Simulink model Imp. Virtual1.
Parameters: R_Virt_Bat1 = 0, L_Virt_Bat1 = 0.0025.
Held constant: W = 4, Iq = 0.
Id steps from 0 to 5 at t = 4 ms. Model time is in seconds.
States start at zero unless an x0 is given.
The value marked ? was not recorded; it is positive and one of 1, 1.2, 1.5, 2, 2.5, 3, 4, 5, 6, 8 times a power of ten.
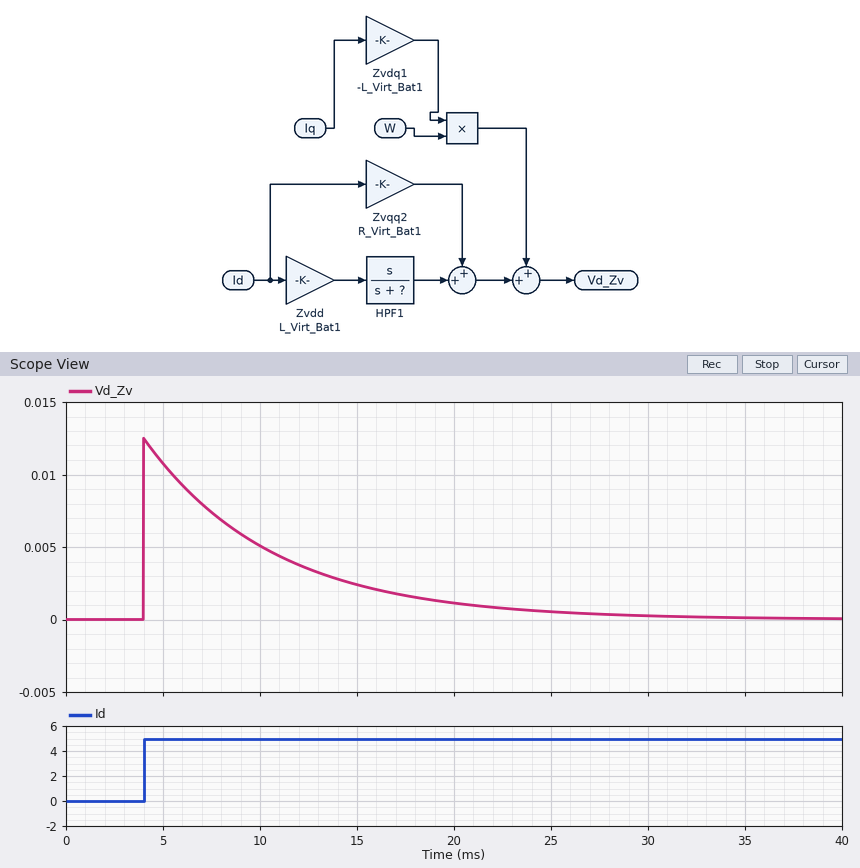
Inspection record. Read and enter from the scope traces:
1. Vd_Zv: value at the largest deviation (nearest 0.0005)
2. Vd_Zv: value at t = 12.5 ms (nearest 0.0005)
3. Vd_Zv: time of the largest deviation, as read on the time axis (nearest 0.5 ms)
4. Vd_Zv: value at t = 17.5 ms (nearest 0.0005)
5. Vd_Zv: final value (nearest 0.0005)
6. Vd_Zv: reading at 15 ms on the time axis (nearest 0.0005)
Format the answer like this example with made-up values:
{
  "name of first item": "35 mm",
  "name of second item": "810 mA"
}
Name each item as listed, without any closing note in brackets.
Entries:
{
  "Vd_Zv: value at the largest deviation": "0.0125",
  "Vd_Zv: value at t = 12.5 ms": "0.0035",
  "Vd_Zv: time of the largest deviation, as read on the time axis": "4.0 ms",
  "Vd_Zv: value at t = 17.5 ms": "0.0015",
  "Vd_Zv: final value": "0.0000",
  "Vd_Zv: reading at 15 ms on the time axis": "0.0025"
}
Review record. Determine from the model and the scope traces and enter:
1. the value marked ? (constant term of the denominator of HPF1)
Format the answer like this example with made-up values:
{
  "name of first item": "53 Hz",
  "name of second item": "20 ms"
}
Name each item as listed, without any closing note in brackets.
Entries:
{
  "the value marked ?": "150"
}
